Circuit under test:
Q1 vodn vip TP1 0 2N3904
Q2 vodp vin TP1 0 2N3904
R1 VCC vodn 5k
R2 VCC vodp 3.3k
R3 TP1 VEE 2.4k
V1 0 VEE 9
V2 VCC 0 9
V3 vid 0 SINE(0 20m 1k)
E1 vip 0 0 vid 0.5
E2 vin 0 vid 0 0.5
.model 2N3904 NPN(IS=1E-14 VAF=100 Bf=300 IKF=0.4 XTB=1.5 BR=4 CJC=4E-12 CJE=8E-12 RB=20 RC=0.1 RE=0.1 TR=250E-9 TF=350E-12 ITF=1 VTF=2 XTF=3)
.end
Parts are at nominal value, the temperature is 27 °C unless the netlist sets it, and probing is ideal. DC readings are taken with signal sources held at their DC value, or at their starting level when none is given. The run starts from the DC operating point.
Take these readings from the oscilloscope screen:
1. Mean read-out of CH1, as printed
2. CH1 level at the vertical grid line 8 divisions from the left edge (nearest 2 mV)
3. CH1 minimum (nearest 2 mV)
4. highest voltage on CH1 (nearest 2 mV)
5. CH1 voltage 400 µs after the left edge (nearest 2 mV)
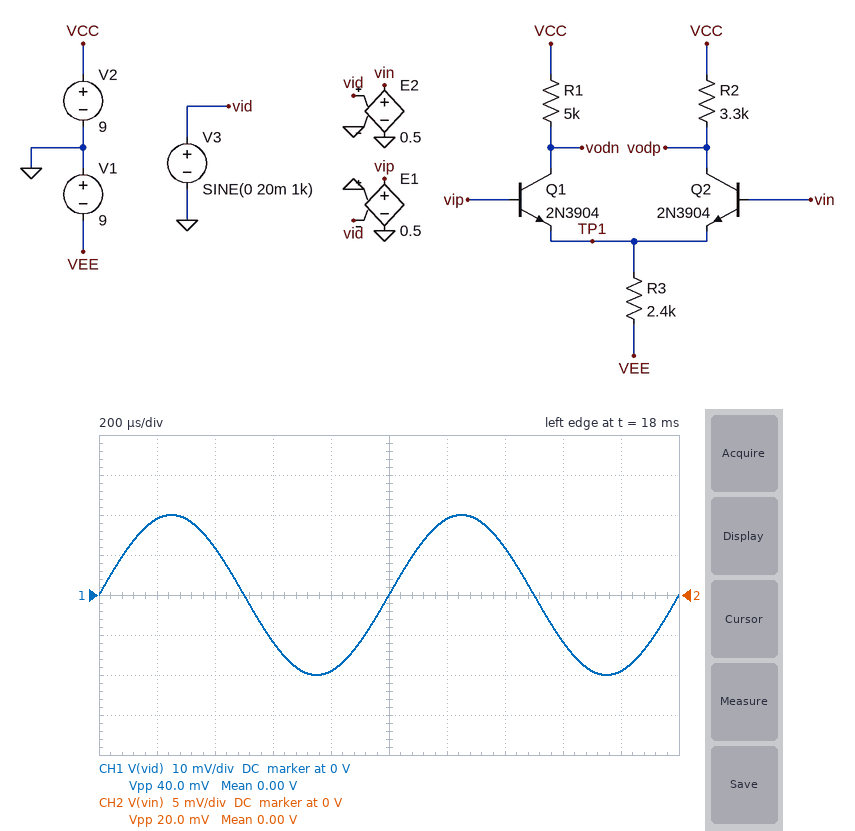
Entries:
0.00 V
-12 mV
-20 mV
20 mV
12 mV
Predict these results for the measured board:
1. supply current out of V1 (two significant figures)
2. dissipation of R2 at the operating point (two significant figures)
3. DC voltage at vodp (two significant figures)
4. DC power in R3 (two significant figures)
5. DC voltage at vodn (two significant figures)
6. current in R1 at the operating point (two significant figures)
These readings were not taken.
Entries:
3.5 mA
10 mW
3.2 V
29 mW
470 mV
1.7 mA
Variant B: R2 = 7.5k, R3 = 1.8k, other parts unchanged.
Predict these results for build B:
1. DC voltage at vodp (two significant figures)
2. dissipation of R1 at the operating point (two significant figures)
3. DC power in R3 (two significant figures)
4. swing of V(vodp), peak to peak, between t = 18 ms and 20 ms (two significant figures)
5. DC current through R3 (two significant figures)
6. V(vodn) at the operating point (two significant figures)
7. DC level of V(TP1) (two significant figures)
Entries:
-700 mV
19 mW
38 mW
4.7 mV
4.6 mA
-690 mV
-710 mV
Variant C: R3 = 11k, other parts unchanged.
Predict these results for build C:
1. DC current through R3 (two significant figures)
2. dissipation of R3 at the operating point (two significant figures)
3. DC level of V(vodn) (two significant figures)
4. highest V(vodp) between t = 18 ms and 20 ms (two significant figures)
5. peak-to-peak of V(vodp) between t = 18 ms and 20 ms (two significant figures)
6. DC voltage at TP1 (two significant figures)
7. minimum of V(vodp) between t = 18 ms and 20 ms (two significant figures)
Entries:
760 µA
6.4 mW
7.1 V
8.2 V
910 mV
-630 mV
7.3 V
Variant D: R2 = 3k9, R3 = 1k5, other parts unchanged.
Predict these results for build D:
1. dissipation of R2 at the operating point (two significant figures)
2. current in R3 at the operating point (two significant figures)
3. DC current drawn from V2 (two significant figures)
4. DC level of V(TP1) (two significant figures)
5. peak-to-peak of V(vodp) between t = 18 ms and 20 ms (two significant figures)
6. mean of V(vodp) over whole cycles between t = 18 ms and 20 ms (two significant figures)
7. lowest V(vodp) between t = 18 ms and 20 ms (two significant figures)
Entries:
24 mW
5.5 mA
4.4 mA
-710 mV
12 mV
-680 mV
-690 mV
